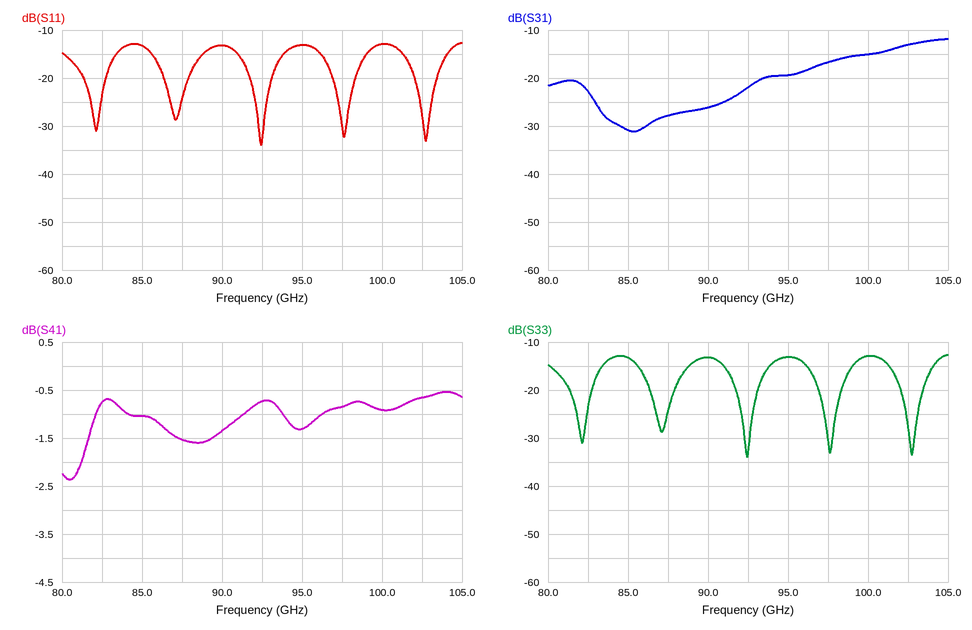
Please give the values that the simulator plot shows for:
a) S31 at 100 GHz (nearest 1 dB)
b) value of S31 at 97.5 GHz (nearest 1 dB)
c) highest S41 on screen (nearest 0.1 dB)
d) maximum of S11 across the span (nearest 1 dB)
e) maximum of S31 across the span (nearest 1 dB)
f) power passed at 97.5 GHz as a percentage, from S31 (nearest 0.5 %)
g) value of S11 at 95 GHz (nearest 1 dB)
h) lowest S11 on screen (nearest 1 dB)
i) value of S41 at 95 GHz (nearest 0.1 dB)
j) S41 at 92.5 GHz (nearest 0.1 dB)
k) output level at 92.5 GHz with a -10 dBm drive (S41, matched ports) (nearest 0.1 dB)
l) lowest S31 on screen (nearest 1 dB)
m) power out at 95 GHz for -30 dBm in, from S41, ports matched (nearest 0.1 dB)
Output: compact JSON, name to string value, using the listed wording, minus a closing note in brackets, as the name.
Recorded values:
{"S31 at 100 GHz": "-15 dB", "value of S31 at 97.5 GHz": "-17 dB", "highest S41 on screen": "-0.5 dB", "maximum of S11 across the span": "-13 dB", "maximum of S31 across the span": "-12 dB", "power passed at 97.5 GHz as a percentage, from S31": "2.0 %", "value of S11 at 95 GHz": "-13 dB", "lowest S11 on screen": "-34 dB", "value of S41 at 95 GHz": "-1.3 dB", "S41 at 92.5 GHz": "-0.7 dB", "output level at 92.5 GHz with a -10 dBm drive (S41, matched ports)": "-10.7 dBm", "lowest S31 on screen": "-31 dB", "power out at 95 GHz for -30 dBm in, from S41, ports matched": "-31.3 dBm"}
